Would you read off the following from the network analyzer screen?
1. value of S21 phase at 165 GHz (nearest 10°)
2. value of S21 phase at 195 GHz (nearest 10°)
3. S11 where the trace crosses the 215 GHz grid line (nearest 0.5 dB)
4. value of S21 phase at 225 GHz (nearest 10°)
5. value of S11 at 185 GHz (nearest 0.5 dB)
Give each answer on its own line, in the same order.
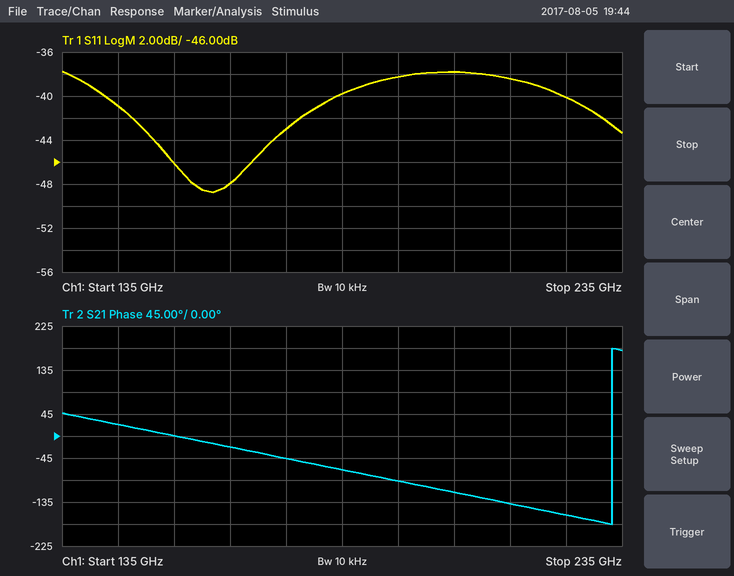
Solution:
-20°
-90°
-38.5 dB
-160°
-40.0 dB
